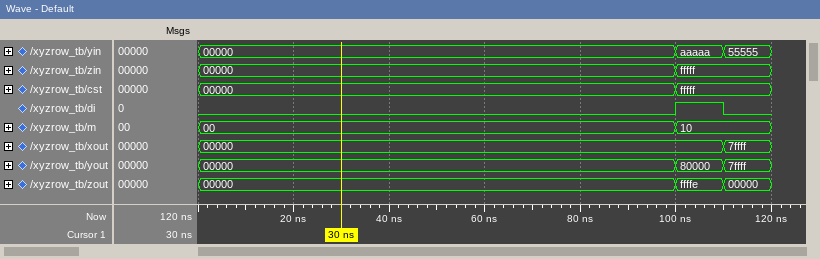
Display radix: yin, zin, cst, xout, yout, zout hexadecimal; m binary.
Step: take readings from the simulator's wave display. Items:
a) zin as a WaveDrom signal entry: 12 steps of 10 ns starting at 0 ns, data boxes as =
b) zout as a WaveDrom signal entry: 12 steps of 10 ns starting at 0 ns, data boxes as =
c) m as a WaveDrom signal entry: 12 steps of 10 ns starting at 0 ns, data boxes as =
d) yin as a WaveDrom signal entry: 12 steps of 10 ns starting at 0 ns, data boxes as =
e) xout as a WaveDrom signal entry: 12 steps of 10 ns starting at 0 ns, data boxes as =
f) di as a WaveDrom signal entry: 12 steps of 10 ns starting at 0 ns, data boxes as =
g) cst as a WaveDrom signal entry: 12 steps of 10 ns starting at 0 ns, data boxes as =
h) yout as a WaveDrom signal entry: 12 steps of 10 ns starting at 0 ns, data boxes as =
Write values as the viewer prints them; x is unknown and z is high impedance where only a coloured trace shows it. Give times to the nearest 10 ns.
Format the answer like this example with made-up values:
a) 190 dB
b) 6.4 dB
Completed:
a) {name: 'zin', wave: '=.........=.', data: '00000 fffff'}
b) {name: 'zout', wave: '=.........==', data: '00000 ffffe 00000'}
c) {name: 'm', wave: '=.........=.', data: '00 10'}
d) {name: 'yin', wave: '=.........==', data: '00000 aaaaa 55555'}
e) {name: 'xout', wave: '=..........=', data: '00000 7ffff'}
f) {name: 'di', wave: '0.........10'}
g) {name: 'cst', wave: '=.........=.', data: '00000 fffff'}
h) {name: 'yout', wave: '=.........==', data: '00000 80000 7ffff'}
